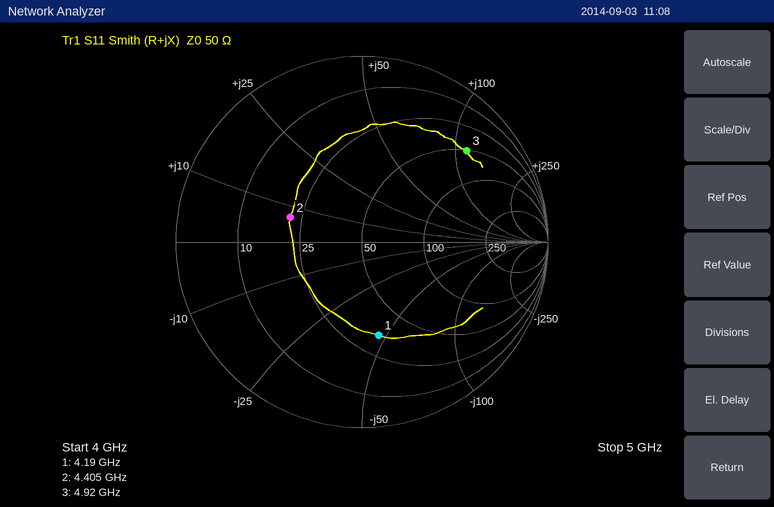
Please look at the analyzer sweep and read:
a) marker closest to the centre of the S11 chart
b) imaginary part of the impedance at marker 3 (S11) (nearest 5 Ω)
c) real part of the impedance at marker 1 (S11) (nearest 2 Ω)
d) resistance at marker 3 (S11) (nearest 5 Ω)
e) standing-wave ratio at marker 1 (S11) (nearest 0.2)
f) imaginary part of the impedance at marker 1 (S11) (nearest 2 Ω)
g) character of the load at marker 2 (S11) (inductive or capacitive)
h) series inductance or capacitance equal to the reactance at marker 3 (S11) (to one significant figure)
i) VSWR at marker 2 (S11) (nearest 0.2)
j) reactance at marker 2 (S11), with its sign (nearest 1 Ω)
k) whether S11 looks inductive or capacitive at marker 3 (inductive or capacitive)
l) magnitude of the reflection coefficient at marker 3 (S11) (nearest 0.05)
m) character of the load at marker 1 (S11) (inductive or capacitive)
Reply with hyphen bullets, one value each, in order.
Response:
- marker 2
- +115 Ω
- 34 Ω
- 50 Ω
- 3.0
- -46 Ω
- inductive
- 4 nH
- 2.4
- +7 Ω
- inductive
- 0.75
- capacitive
